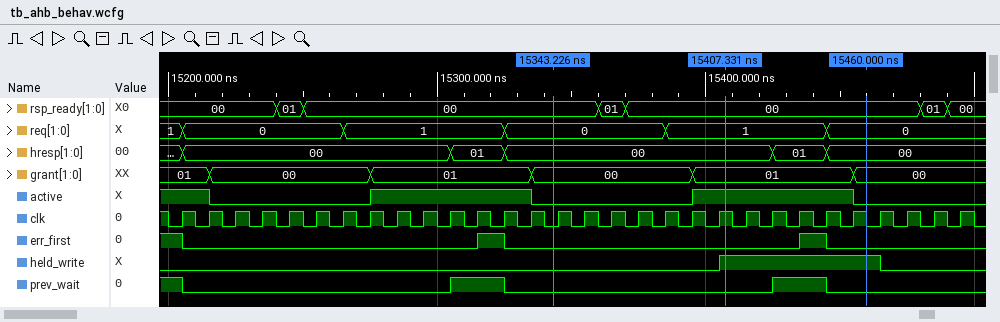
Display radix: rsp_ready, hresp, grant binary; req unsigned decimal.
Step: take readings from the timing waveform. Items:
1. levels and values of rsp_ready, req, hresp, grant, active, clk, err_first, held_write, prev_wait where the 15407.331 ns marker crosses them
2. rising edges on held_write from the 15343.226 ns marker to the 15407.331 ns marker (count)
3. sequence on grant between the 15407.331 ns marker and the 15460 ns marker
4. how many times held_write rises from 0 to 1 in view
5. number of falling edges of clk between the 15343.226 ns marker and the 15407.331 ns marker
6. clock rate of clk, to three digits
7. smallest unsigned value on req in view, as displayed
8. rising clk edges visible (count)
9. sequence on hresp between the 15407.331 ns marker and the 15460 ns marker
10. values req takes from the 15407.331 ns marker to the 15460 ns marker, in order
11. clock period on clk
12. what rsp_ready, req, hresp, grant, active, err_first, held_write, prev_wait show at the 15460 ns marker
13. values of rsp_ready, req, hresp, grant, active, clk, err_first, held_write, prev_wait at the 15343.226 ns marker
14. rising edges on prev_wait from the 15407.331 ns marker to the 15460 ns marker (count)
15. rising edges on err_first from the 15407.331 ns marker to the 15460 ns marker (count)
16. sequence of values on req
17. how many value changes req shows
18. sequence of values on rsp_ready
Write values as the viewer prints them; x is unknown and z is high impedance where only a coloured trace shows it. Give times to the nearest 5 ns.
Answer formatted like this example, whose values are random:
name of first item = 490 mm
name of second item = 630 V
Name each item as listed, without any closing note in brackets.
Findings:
levels and values of rsp_ready, req, hresp, grant, active, clk, err_first, held_write, prev_wait where the 15407.331 ns marker crosses them = rsp_ready=00, req=1, hresp=00, grant=01, active=1, clk=1, err_first=0, held_write=1, prev_wait=0
rising edges on held_write from the 15343.226 ns marker to the 15407.331 ns marker = 1
sequence on grant between the 15407.331 ns marker and the 15460 ns marker = 01, 00
how many times held_write rises from 0 to 1 in view = 1
number of falling edges of clk between the 15343.226 ns marker and the 15407.331 ns marker = 6
clock rate of clk, to three digits = 100 MHz
smallest unsigned value on req in view, as displayed = 0
rising clk edges visible = 30
sequence on hresp between the 15407.331 ns marker and the 15460 ns marker = 00, 01, 00
values req takes from the 15407.331 ns marker to the 15460 ns marker, in order = 1, 0
clock period on clk = 10 ns
what rsp_ready, req, hresp, grant, active, err_first, held_write, prev_wait show at the 15460 ns marker = rsp_ready=00, req=0, hresp=00, grant=00, active=0, err_first=0, held_write=1, prev_wait=0
values of rsp_ready, req, hresp, grant, active, clk, err_first, held_write, prev_wait at the 15343.226 ns marker = rsp_ready=00, req=0, hresp=00, grant=00, active=0, clk=0, err_first=0, held_write=0, prev_wait=0
rising edges on prev_wait from the 15407.331 ns marker to the 15460 ns marker = 1
rising edges on err_first from the 15407.331 ns marker to the 15460 ns marker = 1
sequence of values on req = 1, 0, 1, 0, 1, 0
how many value changes req shows = 5
sequence of values on rsp_ready = 00, 01, 00, 01, 00, 01, 00
